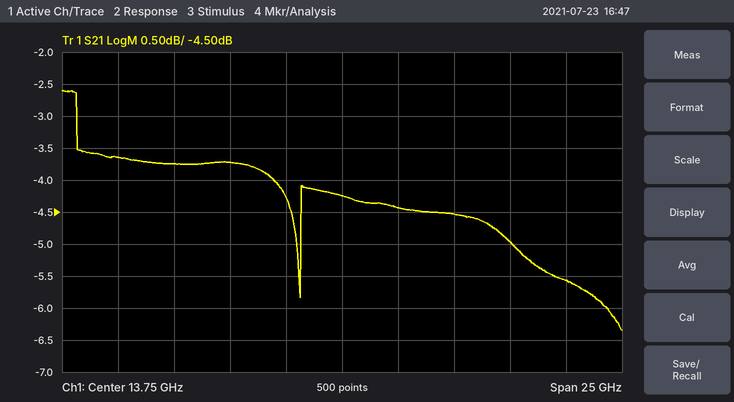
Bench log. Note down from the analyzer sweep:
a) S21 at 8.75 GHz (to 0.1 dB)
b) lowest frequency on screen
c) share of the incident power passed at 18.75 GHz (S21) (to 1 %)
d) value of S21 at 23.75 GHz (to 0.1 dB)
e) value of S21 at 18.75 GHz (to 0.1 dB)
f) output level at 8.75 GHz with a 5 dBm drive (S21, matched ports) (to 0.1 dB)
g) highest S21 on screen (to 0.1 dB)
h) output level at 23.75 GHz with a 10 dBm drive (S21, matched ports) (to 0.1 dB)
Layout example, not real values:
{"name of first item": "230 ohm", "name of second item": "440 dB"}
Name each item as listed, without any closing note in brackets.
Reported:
{"S21 at 8.75 GHz": "-3.7 dB", "lowest frequency on screen": "1.25 GHz", "share of the incident power passed at 18.75 GHz (S21)": "35 %", "value of S21 at 23.75 GHz": "-5.6 dB", "value of S21 at 18.75 GHz": "-4.5 dB", "output level at 8.75 GHz with a 5 dBm drive (S21, matched ports)": "1.3 dBm", "highest S21 on screen": "-2.6 dB", "output level at 23.75 GHz with a 10 dBm drive (S21, matched ports)": "4.4 dBm"}
